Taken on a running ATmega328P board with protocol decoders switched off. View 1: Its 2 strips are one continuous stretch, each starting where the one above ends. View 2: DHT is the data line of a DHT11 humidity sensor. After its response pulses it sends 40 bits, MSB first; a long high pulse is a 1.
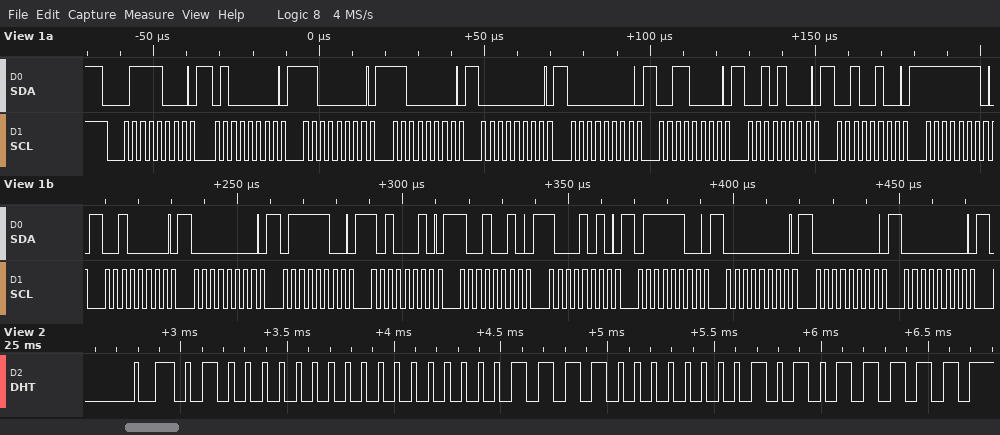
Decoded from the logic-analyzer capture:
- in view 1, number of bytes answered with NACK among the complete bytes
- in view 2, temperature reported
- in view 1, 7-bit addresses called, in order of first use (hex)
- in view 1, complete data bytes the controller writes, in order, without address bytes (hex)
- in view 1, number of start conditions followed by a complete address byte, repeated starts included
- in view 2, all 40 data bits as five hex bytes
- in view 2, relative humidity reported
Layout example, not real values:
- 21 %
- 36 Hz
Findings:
- 0
- 30.1 °C
- 0x3C
- 40 C0 C0 00 00 30 28 24 FE 20 00 7C A2 92 8A 7C 00 00 00
- 1
- 40 00 1E 01 5F
- 64 %
